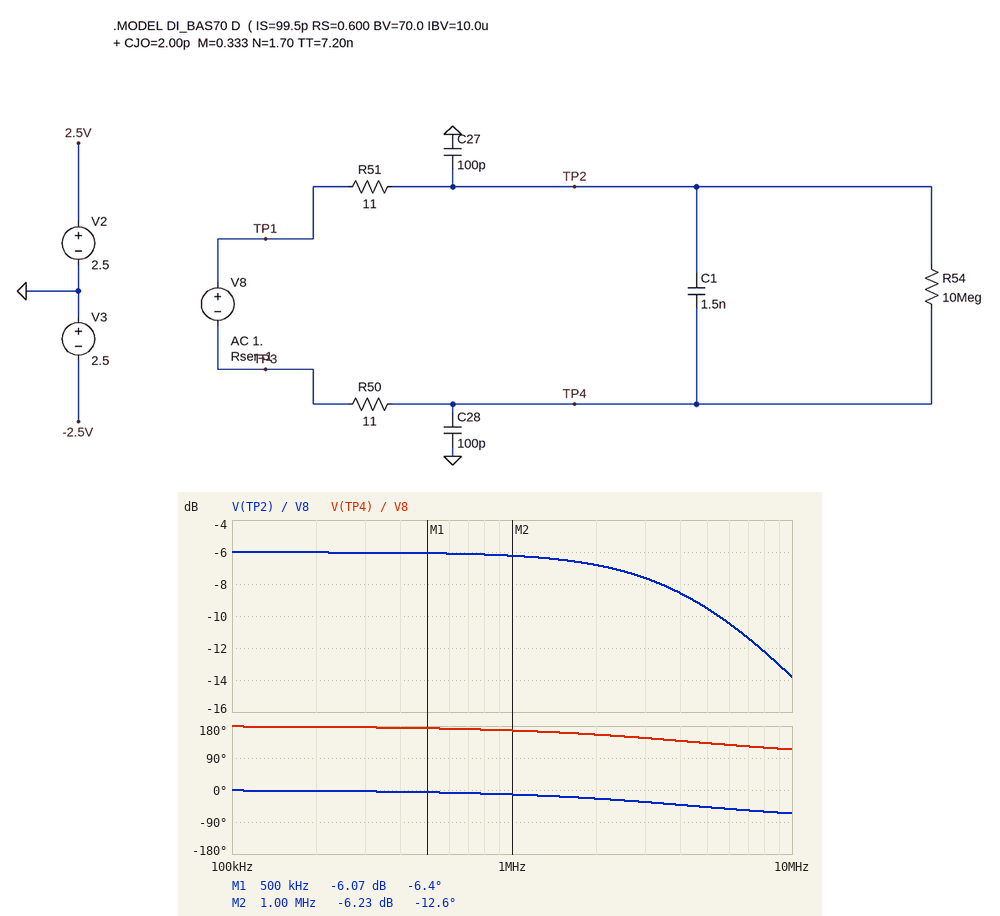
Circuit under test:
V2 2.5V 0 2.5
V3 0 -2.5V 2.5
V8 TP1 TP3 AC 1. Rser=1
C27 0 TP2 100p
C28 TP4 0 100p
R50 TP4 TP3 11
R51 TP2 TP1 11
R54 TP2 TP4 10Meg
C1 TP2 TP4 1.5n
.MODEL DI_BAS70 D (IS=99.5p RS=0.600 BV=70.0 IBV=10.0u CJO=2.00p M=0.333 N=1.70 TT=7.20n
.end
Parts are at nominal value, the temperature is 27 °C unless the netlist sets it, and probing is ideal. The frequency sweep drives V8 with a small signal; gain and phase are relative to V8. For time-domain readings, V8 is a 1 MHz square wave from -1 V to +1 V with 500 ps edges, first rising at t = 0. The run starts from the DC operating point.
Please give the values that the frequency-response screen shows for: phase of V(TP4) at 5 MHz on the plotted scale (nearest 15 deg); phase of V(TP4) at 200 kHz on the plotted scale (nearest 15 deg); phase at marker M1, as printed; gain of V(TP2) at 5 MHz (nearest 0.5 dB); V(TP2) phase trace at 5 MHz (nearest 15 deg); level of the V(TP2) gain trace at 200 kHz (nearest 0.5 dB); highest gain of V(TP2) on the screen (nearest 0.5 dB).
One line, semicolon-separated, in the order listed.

135 deg; 180 deg; -6.4 deg; -9.5 dB; -45 deg; -6.0 dB; -6.0 dB
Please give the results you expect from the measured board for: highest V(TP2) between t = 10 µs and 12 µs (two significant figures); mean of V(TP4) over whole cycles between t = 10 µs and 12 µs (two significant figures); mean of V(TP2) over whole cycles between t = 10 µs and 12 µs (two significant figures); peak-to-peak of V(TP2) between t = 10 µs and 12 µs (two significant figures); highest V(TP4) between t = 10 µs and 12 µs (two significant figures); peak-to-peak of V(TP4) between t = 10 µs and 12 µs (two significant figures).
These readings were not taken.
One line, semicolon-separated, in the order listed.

1.0 V; 500 mV; 500 mV; 1.0 V; 1.0 V; 1.0 V
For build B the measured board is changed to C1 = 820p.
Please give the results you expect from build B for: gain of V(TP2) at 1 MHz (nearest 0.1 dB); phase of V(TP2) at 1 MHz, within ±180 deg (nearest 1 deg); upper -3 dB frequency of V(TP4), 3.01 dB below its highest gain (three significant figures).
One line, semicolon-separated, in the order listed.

-6.1 dB; -7 deg; 7.95 MHz
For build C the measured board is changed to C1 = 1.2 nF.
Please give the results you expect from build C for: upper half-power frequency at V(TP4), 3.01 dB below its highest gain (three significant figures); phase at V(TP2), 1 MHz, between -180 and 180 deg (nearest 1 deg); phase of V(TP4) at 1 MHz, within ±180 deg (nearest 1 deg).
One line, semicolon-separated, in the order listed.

5.54 MHz; -10 deg; 170 deg
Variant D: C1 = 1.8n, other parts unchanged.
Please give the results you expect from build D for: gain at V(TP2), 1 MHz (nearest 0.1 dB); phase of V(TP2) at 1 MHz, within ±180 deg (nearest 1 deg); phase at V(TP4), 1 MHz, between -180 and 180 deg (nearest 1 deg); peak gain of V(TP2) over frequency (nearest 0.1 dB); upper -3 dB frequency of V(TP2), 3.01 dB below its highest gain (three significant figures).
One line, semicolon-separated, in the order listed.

-6.3 dB; -15 deg; 165 deg; -6.0 dB; 3.74 MHz
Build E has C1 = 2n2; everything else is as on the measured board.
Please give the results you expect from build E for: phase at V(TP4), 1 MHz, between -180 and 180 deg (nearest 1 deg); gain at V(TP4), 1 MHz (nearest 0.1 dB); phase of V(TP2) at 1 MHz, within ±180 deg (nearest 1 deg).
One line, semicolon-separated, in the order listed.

162 deg; -6.5 dB; -18 deg
